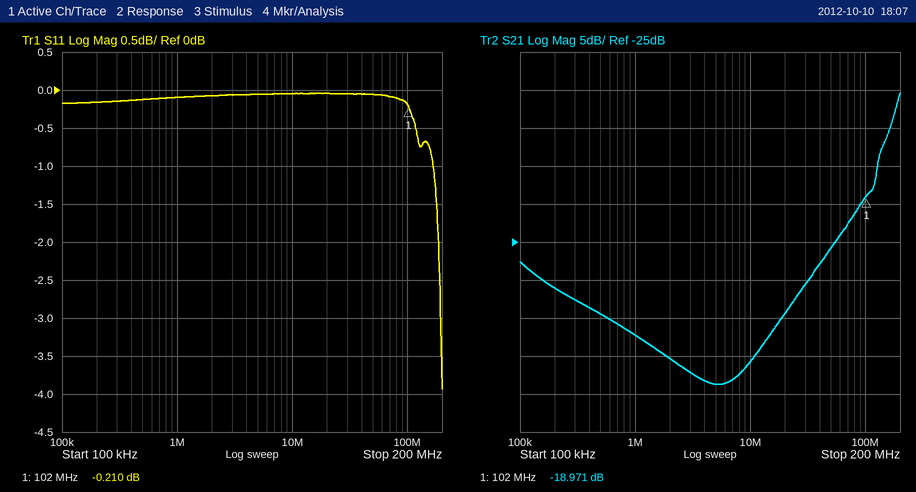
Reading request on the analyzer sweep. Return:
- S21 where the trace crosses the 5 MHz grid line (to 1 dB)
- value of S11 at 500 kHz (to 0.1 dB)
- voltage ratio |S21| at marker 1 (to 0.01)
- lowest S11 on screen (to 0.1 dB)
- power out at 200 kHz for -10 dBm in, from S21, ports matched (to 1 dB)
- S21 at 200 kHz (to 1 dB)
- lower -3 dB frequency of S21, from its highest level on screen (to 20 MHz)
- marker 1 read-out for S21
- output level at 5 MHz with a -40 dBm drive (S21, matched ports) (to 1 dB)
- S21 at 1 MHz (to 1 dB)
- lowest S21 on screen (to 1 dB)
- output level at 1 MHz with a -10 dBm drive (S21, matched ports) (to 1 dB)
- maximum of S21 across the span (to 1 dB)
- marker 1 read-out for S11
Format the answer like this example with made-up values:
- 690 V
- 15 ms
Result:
- -44 dB
- -0.1 dB
- 0.11
- -3.9 dB
- -41 dBm
- -31 dB
- 180 MHz
- -18.971 dB
- -84 dBm
- -37 dB
- -44 dB
- -47 dBm
- -5 dB
- -0.210 dB
